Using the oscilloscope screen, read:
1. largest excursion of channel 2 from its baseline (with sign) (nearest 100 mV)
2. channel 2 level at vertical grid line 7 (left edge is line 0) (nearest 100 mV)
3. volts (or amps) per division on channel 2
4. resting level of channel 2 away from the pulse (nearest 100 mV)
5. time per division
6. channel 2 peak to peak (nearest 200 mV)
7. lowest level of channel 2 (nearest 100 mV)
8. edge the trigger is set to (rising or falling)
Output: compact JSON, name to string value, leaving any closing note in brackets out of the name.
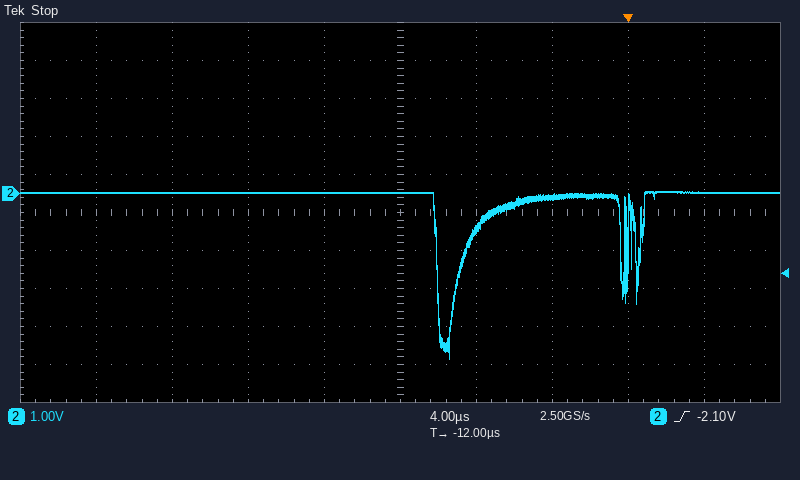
{"largest excursion of channel 2 from its baseline (with sign)": "-4.4 V", "channel 2 level at vertical grid line 7 (left edge is line 0)": "-100 mV", "volts (or amps) per division on channel 2": "1 V", "resting level of channel 2 away from the pulse": "0.0 V", "time per division": "4 µs", "channel 2 peak to peak": "4.4 V", "lowest level of channel 2": "-4.4 V", "edge the trigger is set to": "rising"}
